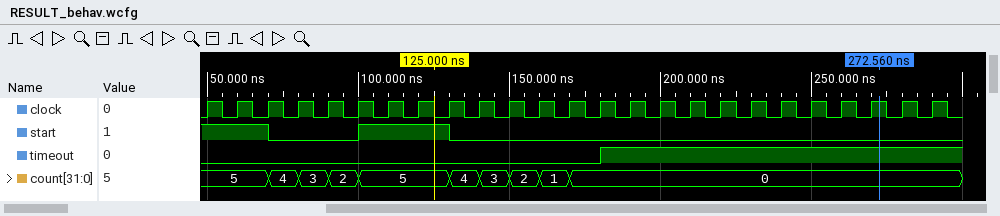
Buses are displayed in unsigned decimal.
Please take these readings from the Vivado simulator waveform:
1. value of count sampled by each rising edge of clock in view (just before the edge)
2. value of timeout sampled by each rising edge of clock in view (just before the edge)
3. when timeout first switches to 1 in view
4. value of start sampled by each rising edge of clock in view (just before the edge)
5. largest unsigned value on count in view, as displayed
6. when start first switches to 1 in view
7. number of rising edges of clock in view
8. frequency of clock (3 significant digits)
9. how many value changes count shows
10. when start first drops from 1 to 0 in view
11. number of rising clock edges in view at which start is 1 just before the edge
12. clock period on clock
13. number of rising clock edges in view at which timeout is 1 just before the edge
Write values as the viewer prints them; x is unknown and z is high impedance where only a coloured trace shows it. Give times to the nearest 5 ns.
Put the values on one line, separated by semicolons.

5, 5, 5, 4, 3, 2, 5, 5, 5, 4, 3, 2, 1, 0, 0, 0, 0, 0, 0, 0, 0, 0, 0, 0, 0; 0 0 0 0 0 0 0 0 0 0 0 0 0 0 1 1 1 1 1 1 1 1 1 1 1; 180 ns; 1 1 1 0 0 0 1 1 1 0 0 0 0 0 0 0 0 0 0 0 0 0 0 0 0; 5; 100 ns; 25; 100 MHz; 9; 70 ns; 6; 10 ns; 11
